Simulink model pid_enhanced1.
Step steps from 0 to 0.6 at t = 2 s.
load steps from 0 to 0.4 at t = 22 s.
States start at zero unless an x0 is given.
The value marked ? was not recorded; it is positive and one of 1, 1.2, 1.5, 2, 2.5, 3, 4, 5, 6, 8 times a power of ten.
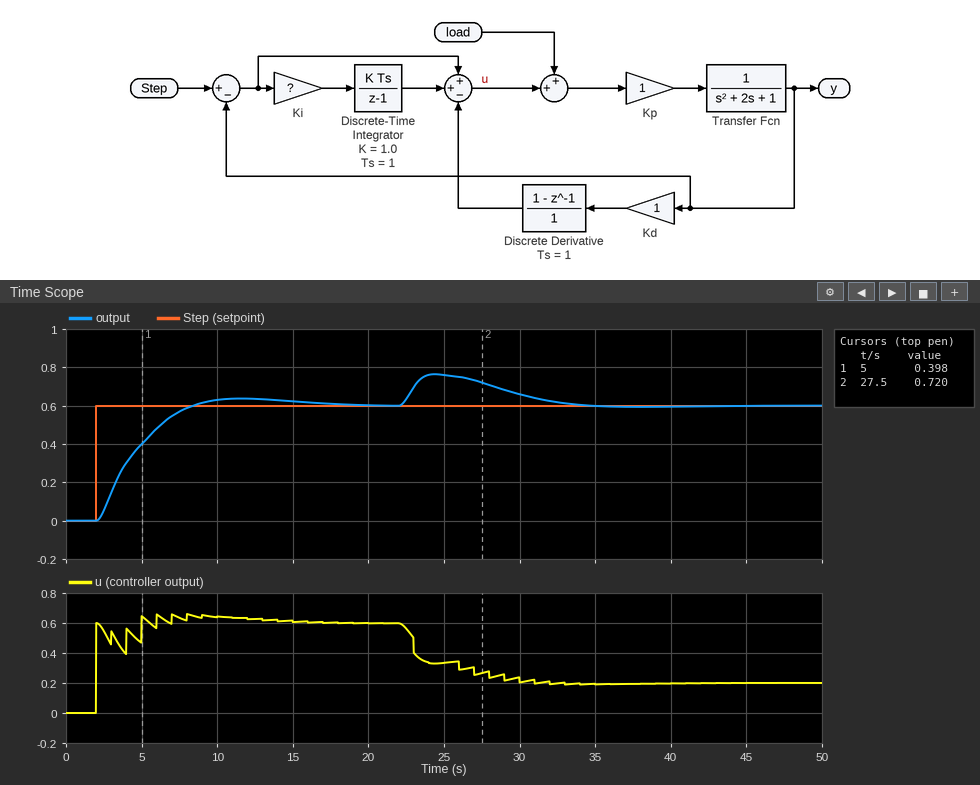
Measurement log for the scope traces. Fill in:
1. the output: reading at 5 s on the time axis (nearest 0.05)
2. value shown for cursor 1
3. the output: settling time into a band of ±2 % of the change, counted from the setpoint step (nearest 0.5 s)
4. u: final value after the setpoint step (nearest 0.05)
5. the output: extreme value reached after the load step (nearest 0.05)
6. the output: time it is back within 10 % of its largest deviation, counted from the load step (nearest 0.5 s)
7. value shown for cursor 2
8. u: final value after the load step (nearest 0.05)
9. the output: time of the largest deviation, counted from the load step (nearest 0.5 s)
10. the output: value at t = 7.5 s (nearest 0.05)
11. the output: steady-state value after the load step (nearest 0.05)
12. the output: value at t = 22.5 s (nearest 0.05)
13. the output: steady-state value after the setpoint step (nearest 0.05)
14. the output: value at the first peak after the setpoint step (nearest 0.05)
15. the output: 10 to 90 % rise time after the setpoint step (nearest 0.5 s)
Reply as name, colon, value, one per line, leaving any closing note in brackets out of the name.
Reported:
the output: reading at 5 s on the time axis: 0.40
value shown for cursor 1: 0.398
the output: settling time into a band of ±2 % of the change, counted from the setpoint step: 15.0 s
u: final value after the setpoint step: 0.60
the output: extreme value reached after the load step: 0.75
the output: time it is back within 10 % of its largest deviation, counted from the load step: 10.5 s
value shown for cursor 2: 0.720
u: final value after the load step: 0.20
the output: time of the largest deviation, counted from the load step: 2.5 s
the output: value at t = 7.5 s: 0.55
the output: steady-state value after the load step: 0.60
the output: value at t = 22.5 s: 0.65
the output: steady-state value after the setpoint step: 0.60
the output: value at the first peak after the setpoint step: 0.65
the output: 10 to 90 % rise time after the setpoint step: 4.5 s
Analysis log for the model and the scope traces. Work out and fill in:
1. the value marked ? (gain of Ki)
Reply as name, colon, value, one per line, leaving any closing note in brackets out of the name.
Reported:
the value marked ?: 0.4
